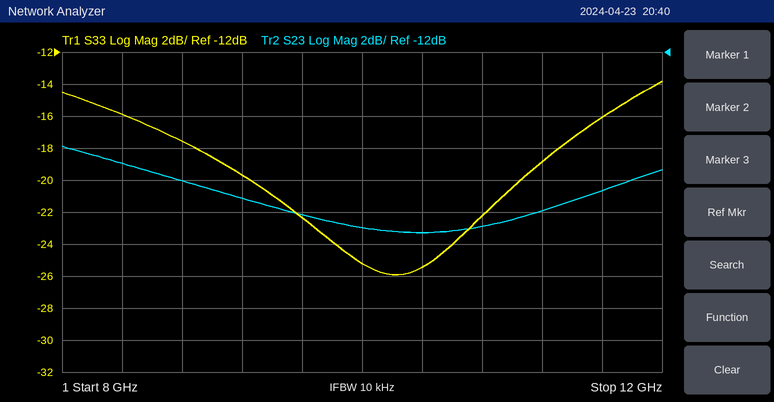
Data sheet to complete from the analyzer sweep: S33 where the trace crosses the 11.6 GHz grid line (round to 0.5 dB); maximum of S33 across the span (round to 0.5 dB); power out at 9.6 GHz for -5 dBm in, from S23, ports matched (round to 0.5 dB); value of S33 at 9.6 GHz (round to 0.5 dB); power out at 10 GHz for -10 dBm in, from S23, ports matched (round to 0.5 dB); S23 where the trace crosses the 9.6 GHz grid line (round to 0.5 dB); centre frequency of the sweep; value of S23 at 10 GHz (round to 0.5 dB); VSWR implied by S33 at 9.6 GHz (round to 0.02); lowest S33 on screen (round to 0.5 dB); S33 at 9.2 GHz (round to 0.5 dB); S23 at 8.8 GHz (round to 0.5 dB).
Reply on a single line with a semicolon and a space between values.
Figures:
-16.0 dB; -14.0 dB; -27.0 dBm; -22.5 dB; -33.0 dBm; -22.0 dB; 10 GHz; -23.0 dB; 1.16; -26.0 dB; -19.5 dB; -20.0 dB
